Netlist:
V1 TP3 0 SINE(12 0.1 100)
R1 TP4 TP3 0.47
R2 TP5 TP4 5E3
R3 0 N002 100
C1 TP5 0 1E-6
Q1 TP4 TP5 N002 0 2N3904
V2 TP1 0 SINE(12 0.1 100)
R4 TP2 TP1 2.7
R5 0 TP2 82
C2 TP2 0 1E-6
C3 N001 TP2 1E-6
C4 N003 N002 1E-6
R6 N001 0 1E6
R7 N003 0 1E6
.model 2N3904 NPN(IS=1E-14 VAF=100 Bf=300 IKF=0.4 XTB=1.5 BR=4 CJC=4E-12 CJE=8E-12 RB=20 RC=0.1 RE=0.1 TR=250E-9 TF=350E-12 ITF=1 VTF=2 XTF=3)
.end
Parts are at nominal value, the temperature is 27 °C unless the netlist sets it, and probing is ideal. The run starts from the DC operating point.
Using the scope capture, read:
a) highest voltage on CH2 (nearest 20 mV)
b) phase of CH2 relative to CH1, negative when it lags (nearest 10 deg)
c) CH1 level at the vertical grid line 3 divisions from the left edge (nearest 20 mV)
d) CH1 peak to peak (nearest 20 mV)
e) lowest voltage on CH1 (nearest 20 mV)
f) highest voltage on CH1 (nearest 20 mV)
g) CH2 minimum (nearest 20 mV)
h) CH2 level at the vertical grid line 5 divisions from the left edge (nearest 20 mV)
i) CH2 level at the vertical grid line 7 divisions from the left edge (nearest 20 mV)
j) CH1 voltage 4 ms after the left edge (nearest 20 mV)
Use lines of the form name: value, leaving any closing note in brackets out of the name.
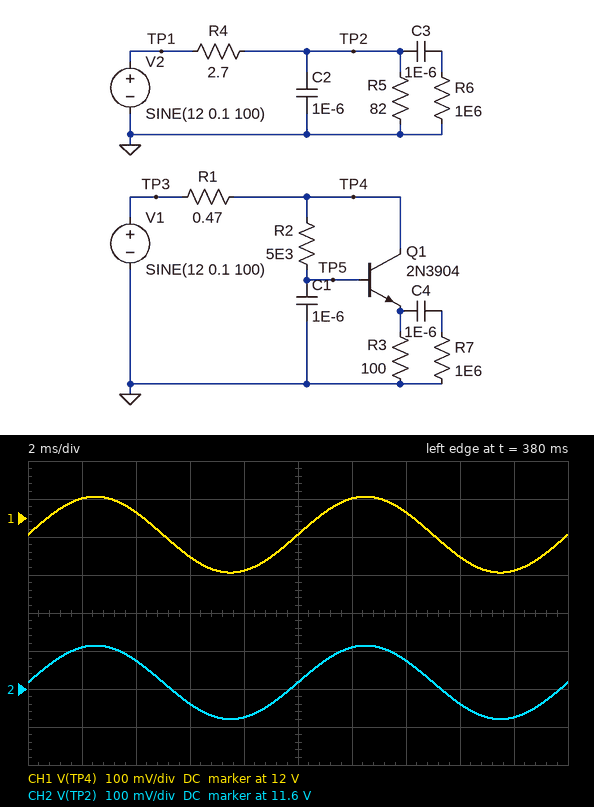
highest voltage on CH2: 11.72 V
phase of CH2 relative to CH1, negative when it lags: 0 deg
CH1 level at the vertical grid line 3 divisions from the left edge: 11.90 V
CH1 peak to peak: 200 mV
lowest voltage on CH1: 11.86 V
highest voltage on CH1: 12.06 V
CH2 minimum: 11.52 V
CH2 level at the vertical grid line 5 divisions from the left edge: 11.62 V
CH2 level at the vertical grid line 7 divisions from the left edge: 11.68 V
CH1 voltage 4 ms after the left edge: 12.02 V
